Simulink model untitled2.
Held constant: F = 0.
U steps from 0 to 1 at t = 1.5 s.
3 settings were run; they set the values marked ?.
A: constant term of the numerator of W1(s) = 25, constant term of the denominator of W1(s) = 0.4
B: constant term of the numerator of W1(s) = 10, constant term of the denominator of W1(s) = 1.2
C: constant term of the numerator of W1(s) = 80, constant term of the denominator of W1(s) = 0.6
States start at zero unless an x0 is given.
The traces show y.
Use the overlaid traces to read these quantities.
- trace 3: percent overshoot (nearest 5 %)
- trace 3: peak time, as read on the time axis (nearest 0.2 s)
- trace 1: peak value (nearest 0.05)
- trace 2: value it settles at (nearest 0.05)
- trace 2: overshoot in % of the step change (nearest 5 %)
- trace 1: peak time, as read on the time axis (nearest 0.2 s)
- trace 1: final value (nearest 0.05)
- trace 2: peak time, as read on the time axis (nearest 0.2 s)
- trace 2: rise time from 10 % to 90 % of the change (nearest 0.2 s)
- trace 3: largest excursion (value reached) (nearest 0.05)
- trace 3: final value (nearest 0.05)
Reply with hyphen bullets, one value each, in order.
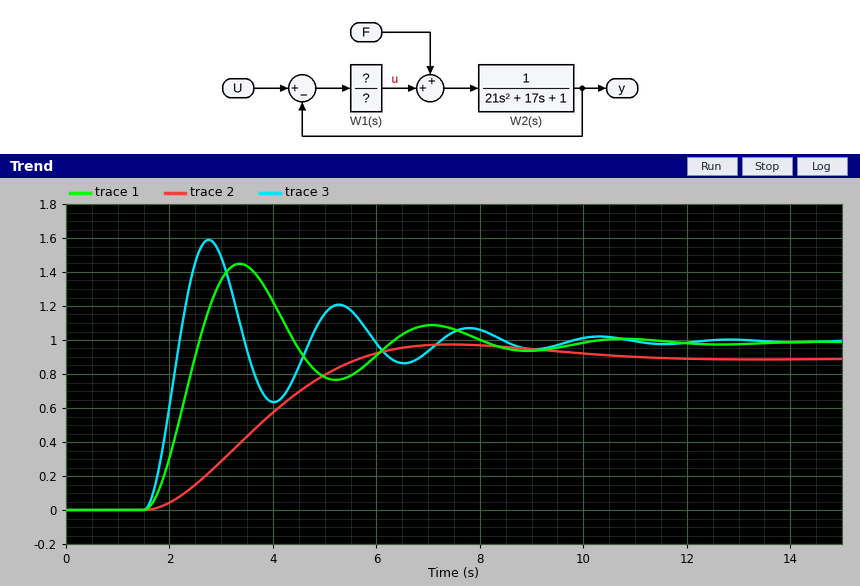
- 60 %
- 2.8 s
- 1.45
- 0.90
- 10 %
- 3.4 s
- 1.00
- 7.4 s
- 2.8 s
- 1.60
- 1.00
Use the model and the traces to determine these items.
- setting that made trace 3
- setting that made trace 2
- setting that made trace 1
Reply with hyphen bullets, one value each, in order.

- C
- B
- A
